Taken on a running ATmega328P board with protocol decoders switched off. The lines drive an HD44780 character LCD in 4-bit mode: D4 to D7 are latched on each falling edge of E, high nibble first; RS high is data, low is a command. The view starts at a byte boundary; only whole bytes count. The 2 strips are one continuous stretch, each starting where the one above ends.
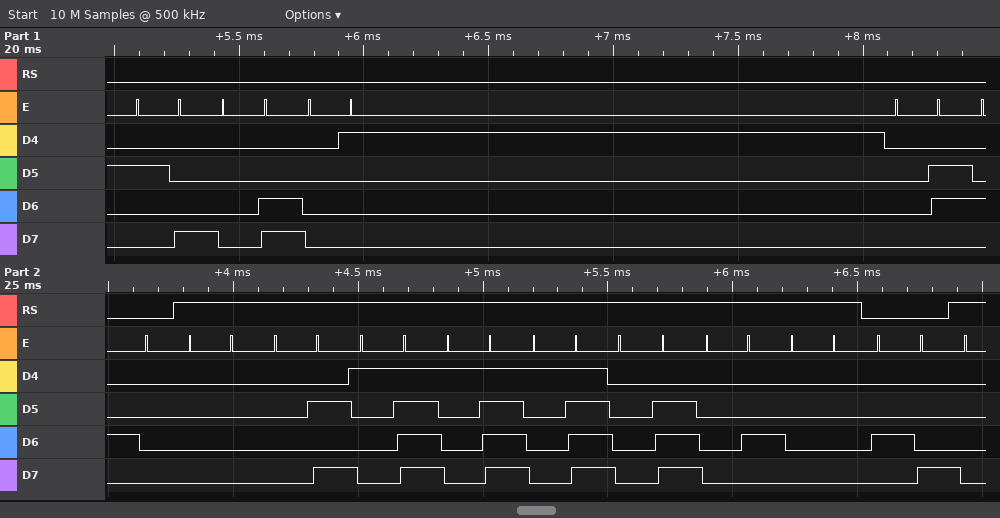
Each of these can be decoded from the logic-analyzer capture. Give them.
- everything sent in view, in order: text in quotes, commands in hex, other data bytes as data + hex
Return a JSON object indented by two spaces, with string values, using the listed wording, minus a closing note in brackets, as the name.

{
  "everything sent in view, in order: text in quotes, commands in hex, other data bytes as data + hex": "0x28 0x0C 0x01 0x06 0x40 data 00 0A 1F 1F 1F 0E 04 00 0x48"
}
